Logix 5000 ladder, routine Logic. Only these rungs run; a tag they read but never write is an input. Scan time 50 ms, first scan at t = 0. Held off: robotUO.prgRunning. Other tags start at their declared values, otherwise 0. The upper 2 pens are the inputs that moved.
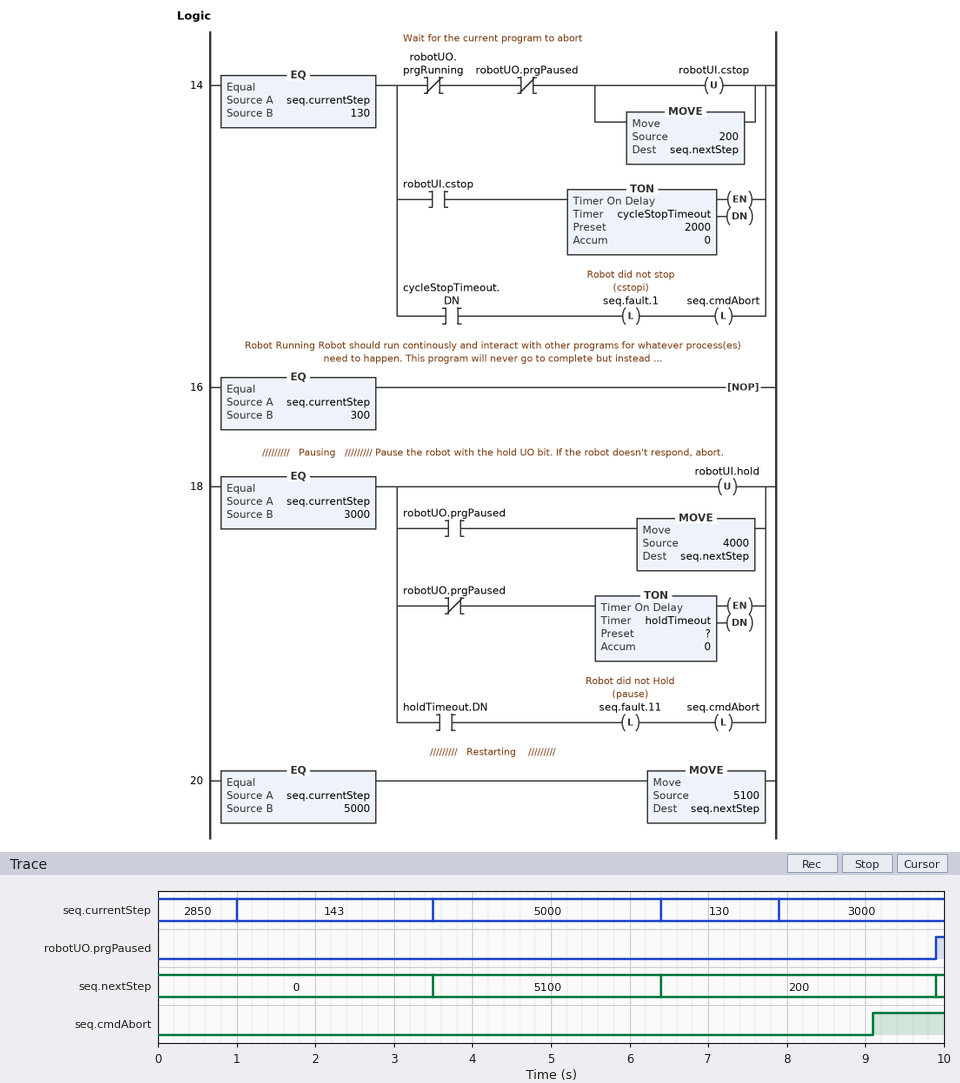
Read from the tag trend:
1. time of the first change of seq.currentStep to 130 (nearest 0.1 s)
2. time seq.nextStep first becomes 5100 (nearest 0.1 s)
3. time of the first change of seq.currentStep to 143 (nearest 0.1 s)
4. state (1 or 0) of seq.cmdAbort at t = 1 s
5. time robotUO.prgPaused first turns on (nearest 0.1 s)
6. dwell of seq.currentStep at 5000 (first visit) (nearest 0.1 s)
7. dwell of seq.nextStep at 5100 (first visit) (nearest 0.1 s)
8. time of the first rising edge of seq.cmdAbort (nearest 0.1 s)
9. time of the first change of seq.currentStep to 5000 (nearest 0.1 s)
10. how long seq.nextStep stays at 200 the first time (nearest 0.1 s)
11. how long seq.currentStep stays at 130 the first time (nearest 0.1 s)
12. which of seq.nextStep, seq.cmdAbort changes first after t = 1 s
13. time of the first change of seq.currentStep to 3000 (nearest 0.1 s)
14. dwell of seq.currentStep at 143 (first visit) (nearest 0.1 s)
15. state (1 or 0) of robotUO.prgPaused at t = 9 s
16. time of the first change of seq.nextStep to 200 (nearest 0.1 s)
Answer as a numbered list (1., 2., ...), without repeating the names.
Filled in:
1. 6.4 s
2. 3.5 s
3. 1.0 s
4. 0
5. 9.9 s
6. 2.9 s
7. 2.9 s
8. 9.1 s
9. 3.5 s
10. 3.5 s
11. 1.5 s
12. seq.nextStep
13. 7.9 s
14. 2.5 s
15. 0
16. 6.4 s
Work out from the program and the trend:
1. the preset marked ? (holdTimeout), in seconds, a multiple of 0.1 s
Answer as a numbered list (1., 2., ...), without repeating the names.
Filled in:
1. 1.2 s
